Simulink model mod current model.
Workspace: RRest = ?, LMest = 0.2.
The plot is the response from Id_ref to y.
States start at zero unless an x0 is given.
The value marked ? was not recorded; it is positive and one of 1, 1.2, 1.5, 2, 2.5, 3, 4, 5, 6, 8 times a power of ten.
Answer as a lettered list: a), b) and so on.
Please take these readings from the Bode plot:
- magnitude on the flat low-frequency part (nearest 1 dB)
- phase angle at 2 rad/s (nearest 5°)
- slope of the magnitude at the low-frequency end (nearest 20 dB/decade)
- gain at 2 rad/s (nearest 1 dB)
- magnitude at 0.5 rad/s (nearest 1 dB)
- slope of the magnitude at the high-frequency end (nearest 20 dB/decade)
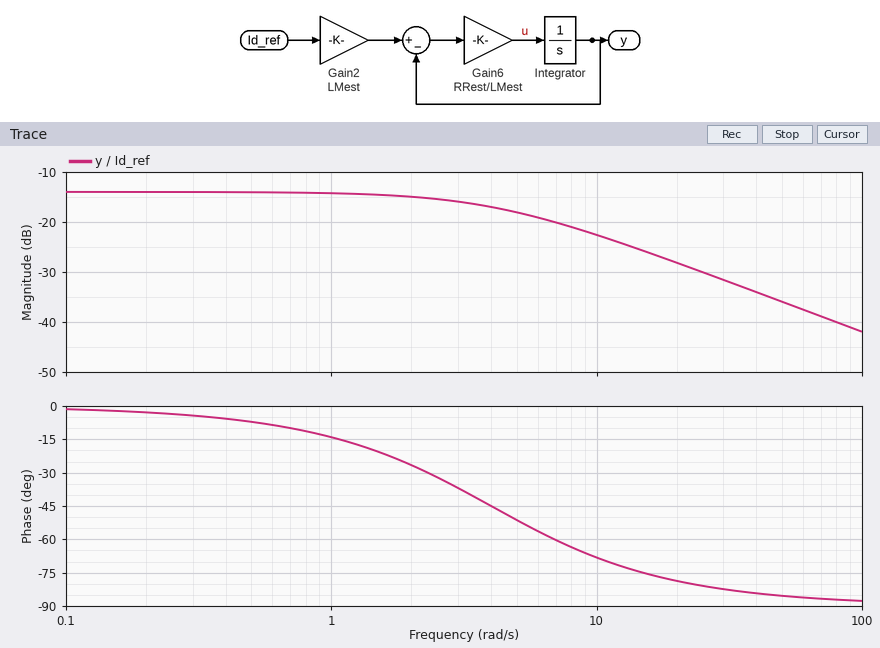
a) -14 dB
b) -25°
c) 0 dB/decade
d) -15 dB
e) -14 dB
f) -20 dB/decade
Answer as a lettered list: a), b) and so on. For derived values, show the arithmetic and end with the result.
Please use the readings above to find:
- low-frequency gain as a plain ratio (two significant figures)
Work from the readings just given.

a) 10^(-14 / 20) = 0.20
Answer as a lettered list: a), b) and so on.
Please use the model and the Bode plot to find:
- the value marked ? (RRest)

a) 0.8
